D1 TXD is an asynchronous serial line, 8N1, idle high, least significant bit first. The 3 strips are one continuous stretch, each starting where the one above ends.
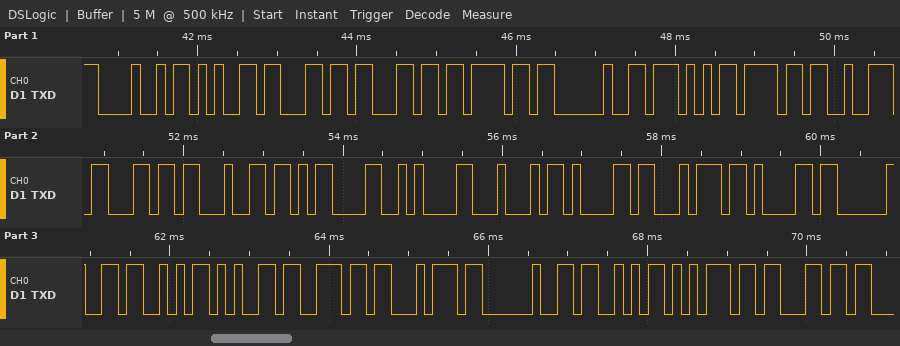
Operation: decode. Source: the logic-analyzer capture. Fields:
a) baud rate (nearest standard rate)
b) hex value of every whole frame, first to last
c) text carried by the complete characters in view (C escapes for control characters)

9600 baud
0x48 0x65 0x6C 0x6C 0x6F 0x20 0x57 0x6F 0x72 0x6C 0x64 0x0D 0x0A 0x44 0x61 0x74 0x61 0x20 0x53 0x65 0x6E 0x74 0x20 0x53 0x75 0x63
"Hello World\r\nData Sent Suc"
